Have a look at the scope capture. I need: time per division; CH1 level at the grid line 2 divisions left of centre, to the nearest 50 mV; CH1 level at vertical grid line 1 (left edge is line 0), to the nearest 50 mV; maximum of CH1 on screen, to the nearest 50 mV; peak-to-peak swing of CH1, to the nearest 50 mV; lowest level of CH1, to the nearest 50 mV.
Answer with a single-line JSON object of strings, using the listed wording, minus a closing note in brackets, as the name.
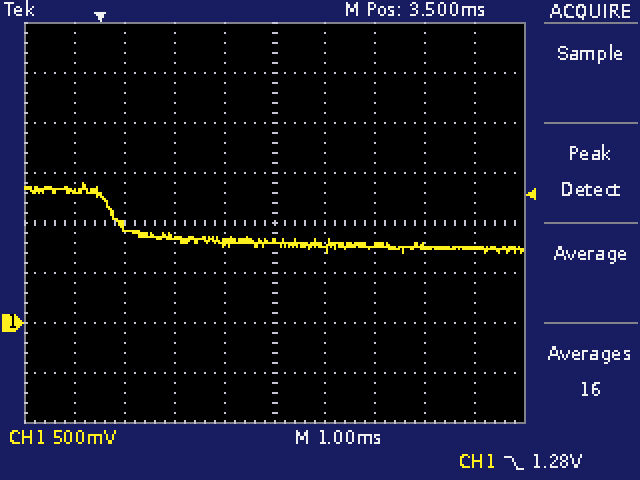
{"time per division": "1 ms", "CH1 level at the grid line 2 divisions left of centre, to the nearest 50 mV": "850 mV", "CH1 level at vertical grid line 1 (left edge is line 0), to the nearest 50 mV": "1.30 V", "maximum of CH1 on screen, to the nearest 50 mV": "1.40 V", "peak-to-peak swing of CH1, to the nearest 50 mV": "700 mV", "lowest level of CH1, to the nearest 50 mV": "700 mV"}
